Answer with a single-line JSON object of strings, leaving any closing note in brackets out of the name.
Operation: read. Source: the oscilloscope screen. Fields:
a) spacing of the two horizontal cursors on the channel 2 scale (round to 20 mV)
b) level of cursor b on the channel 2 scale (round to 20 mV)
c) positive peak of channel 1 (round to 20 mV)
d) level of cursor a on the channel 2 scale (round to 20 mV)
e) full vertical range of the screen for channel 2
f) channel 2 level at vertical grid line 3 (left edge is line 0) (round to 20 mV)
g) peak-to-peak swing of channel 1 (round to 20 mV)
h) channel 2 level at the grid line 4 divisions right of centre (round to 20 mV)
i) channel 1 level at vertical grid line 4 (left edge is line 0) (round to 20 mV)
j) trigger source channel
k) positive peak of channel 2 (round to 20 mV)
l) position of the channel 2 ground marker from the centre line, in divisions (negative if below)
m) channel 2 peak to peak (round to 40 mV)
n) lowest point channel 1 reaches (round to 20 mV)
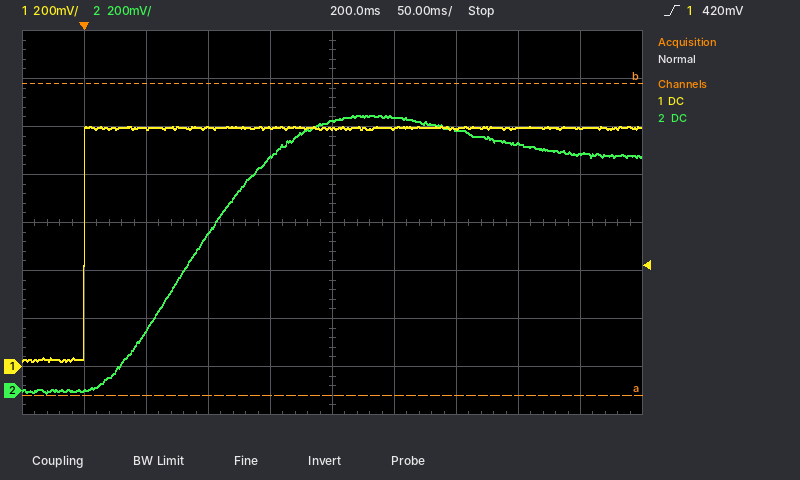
{"spacing of the two horizontal cursors on the channel 2 scale": "1.30 V", "level of cursor b on the channel 2 scale": "1.28 V", "positive peak of channel 1": "1.00 V", "level of cursor a on the channel 2 scale": "-20 mV", "full vertical range of the screen for channel 2": "1.6 V", "channel 2 level at vertical grid line 3 (left edge is line 0)": "660 mV", "peak-to-peak swing of channel 1": "980 mV", "channel 2 level at the grid line 4 divisions right of centre": "980 mV", "channel 1 level at vertical grid line 4 (left edge is line 0)": "1.00 V", "trigger source channel": "channel 1", "positive peak of channel 2": "1.14 V", "position of the channel 2 ground marker from the centre line, in divisions": "-3.5 div", "channel 2 peak to peak": "1.16 V", "lowest point channel 1 reaches": "20 mV"}
